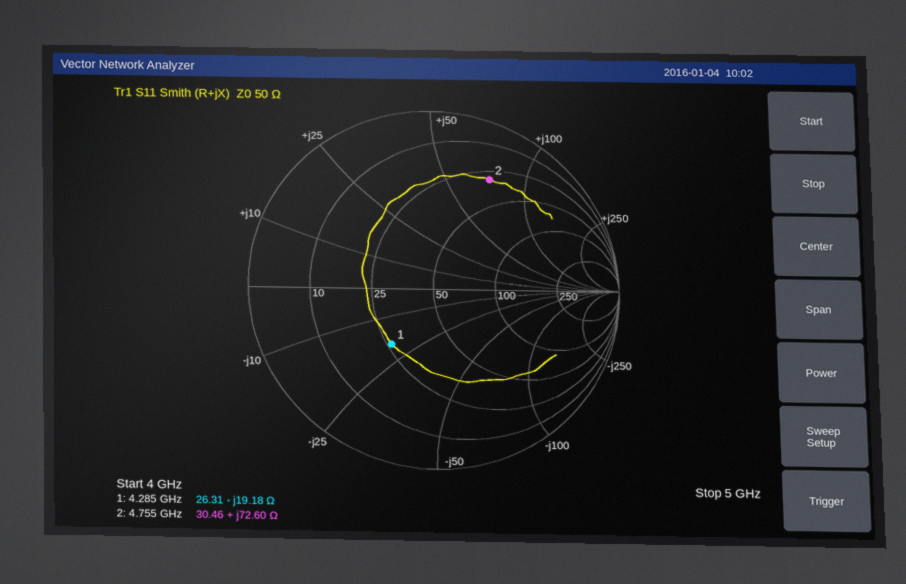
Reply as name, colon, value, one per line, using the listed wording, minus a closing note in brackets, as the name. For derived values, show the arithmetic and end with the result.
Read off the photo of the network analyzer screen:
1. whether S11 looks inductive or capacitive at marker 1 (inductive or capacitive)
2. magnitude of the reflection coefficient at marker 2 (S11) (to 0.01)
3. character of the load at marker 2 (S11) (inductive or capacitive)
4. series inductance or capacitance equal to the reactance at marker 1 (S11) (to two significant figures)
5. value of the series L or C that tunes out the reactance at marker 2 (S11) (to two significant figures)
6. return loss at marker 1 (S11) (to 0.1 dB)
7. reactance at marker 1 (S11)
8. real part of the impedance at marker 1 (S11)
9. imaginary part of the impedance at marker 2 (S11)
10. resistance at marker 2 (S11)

whether S11 looks inductive or capacitive at marker 1: capacitive
magnitude of the reflection coefficient at marker 2 (S11): 0.69
character of the load at marker 2 (S11): inductive
series inductance or capacitance equal to the reactance at marker 1 (S11): C = 1/(2π × 4.285 GHz × 19.18 Ω) ≈ 1.9 pF
value of the series L or C that tunes out the reactance at marker 2 (S11): C = 1/(2π × 4.755 GHz × 72.6 Ω) ≈ 461 fF, so 460 fF to two significant figures
return loss at marker 1 (S11): 8.2 dB
reactance at marker 1: -19.18 Ω
real part of the impedance at marker 1: 26.31 Ω
imaginary part of the impedance at marker 2: +72.60 Ω
resistance at marker 2: 30.46 Ω
